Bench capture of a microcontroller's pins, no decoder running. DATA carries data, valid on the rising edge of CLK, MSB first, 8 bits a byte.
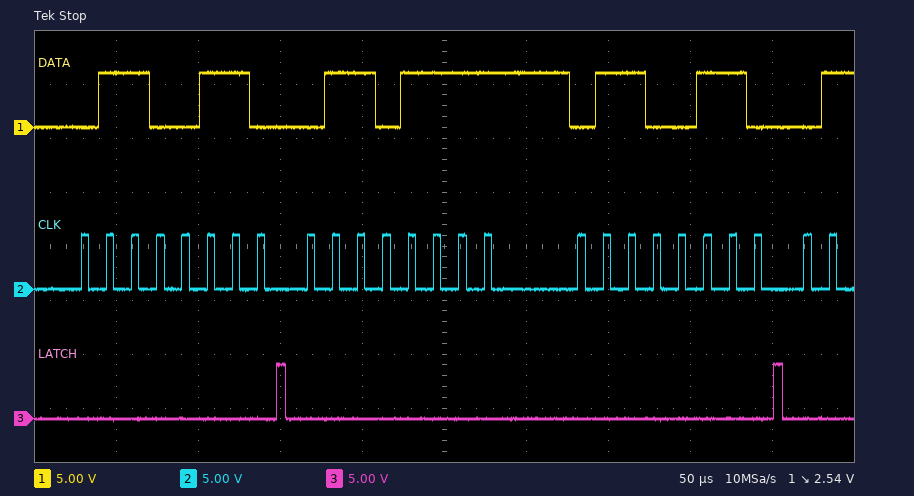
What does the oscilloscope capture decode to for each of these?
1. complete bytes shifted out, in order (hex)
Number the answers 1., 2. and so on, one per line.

1. 66 6F 66
